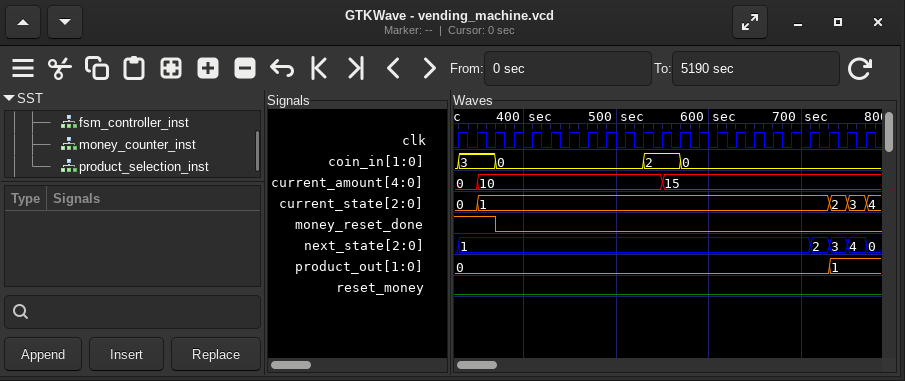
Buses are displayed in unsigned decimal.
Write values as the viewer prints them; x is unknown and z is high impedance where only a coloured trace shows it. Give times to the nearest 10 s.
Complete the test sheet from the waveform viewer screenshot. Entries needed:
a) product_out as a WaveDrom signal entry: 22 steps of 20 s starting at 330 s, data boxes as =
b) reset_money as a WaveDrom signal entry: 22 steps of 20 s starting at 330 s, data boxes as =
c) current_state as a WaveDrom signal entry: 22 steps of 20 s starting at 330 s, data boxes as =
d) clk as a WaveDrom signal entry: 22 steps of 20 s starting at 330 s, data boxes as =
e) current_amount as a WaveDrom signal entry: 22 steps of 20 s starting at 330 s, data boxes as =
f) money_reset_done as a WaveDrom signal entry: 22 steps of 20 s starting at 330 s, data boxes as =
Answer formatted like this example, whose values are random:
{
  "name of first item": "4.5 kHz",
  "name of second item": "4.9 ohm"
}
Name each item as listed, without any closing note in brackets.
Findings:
{
  "product_out as a WaveDrom signal entry: 22 steps of 20 s starting at 330 s, data boxes as =": "{name: 'product_out', wave: '=...................=.', data: '0 1'}",
  "reset_money as a WaveDrom signal entry: 22 steps of 20 s starting at 330 s, data boxes as =": "{name: 'reset_money', wave: '0.....................'}",
  "current_state as a WaveDrom signal entry: 22 steps of 20 s starting at 330 s, data boxes as =": "{name: 'current_state', wave: '==..................==', data: '0 1 2 3'}",
  "clk as a WaveDrom signal entry: 22 steps of 20 s starting at 330 s, data boxes as =": "{name: 'clk', wave: 'p.....................'}",
  "current_amount as a WaveDrom signal entry: 22 steps of 20 s starting at 330 s, data boxes as =": "{name: 'current_amount', wave: '==.........=..........', data: '0 10 15'}",
  "money_reset_done as a WaveDrom signal entry: 22 steps of 20 s starting at 330 s, data boxes as =": "{name: 'money_reset_done', wave: '1.0...................'}"
}
